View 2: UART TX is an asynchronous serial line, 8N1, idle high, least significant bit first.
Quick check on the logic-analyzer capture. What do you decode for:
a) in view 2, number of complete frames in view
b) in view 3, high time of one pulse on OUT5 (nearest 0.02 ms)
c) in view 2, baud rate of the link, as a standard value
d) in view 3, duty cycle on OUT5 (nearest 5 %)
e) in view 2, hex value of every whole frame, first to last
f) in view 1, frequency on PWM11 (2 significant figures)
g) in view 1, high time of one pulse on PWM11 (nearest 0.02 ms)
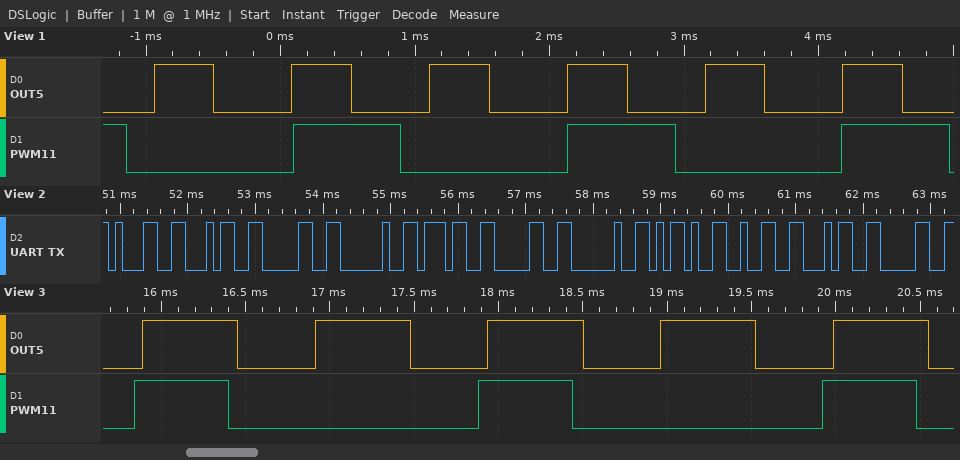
11
0.56 ms
9600 baud
55 %
31 34 30 20 37 30 20 2D 32 34 30
490 Hz
0.80 ms
